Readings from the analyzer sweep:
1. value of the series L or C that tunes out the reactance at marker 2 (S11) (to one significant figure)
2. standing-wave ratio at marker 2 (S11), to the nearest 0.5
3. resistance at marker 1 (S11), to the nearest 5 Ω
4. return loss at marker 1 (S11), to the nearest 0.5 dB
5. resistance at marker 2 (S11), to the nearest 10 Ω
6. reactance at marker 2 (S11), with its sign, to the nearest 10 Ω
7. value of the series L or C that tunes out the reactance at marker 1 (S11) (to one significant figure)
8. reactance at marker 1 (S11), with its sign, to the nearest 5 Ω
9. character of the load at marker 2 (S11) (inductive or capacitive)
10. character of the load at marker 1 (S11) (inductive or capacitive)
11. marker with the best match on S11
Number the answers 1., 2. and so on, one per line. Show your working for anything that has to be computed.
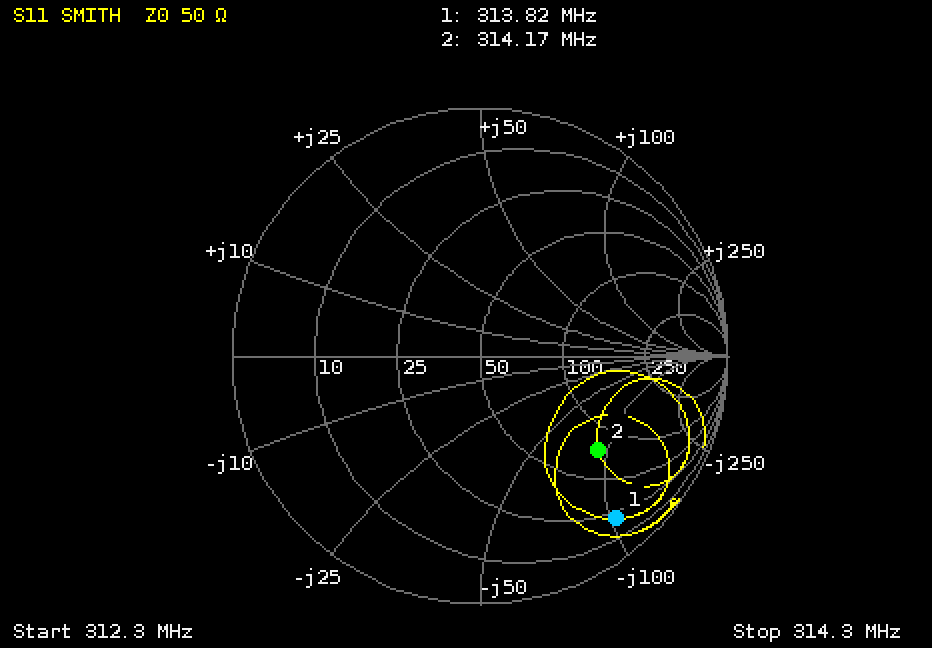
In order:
1. L = 90 Ω/(2π × 314.17 MHz) ≈ 45.6 nH, so 50 nH to one significant figure
2. 4.0
3. 20 Ω
4. 1.5 dB
5. 80 Ω
6. -90 Ω
7. L = 105 Ω/(2π × 313.82 MHz) ≈ 53.3 nH, so 50 nH to one significant figure
8. -105 Ω
9. capacitive
10. capacitive
11. marker 2
